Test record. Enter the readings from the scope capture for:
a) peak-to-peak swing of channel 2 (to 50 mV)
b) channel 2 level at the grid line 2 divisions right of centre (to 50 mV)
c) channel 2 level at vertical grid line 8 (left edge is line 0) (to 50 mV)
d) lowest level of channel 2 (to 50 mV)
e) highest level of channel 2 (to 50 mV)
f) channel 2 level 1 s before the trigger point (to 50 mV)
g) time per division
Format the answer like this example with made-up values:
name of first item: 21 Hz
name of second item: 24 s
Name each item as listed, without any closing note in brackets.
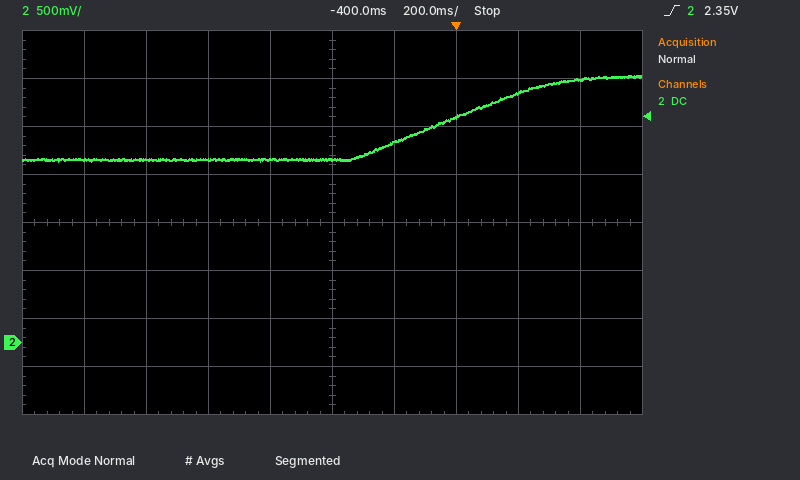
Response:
peak-to-peak swing of channel 2: 900 mV
channel 2 level at the grid line 2 divisions right of centre: 2.35 V
channel 2 level at vertical grid line 8 (left edge is line 0): 2.60 V
lowest level of channel 2: 1.90 V
highest level of channel 2: 2.80 V
channel 2 level 1 s before the trigger point: 1.90 V
time per division: 200 ms
